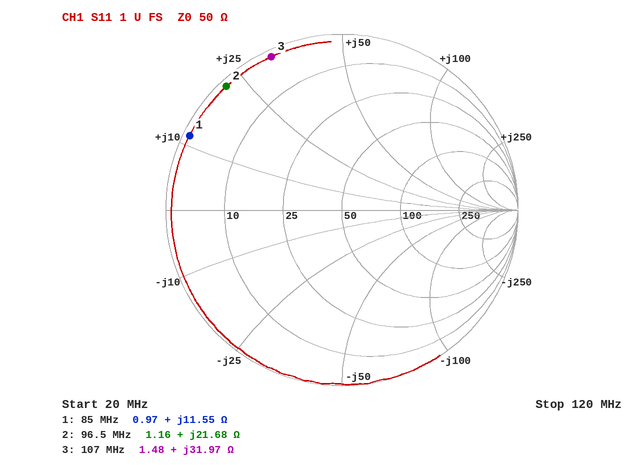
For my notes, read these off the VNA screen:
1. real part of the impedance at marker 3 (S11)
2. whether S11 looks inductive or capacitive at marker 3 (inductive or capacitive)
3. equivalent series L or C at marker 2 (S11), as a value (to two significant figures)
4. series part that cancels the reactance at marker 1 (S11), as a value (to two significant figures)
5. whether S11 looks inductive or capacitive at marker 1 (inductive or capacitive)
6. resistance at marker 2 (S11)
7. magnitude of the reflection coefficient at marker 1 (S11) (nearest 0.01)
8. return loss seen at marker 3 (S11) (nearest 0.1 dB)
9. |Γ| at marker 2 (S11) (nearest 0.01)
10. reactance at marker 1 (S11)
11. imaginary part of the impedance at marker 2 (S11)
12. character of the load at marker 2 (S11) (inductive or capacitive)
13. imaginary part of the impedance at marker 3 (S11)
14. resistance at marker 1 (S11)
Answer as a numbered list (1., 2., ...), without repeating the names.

1. 1.48 Ω
2. inductive
3. 36 nH
4. 160 pF
5. inductive
6. 1.16 Ω
7. 0.96
8. 0.4 dB
9. 0.96
10. +11.55 Ω
11. +21.68 Ω
12. inductive
13. +31.97 Ω
14. 0.97 Ω
